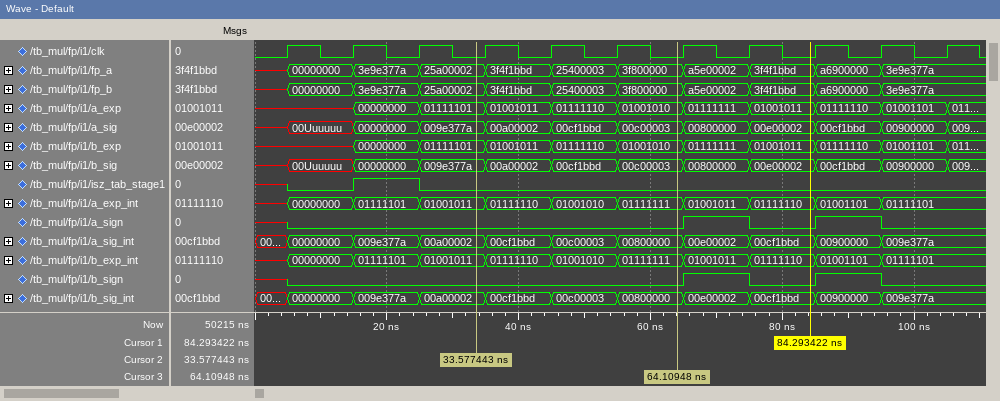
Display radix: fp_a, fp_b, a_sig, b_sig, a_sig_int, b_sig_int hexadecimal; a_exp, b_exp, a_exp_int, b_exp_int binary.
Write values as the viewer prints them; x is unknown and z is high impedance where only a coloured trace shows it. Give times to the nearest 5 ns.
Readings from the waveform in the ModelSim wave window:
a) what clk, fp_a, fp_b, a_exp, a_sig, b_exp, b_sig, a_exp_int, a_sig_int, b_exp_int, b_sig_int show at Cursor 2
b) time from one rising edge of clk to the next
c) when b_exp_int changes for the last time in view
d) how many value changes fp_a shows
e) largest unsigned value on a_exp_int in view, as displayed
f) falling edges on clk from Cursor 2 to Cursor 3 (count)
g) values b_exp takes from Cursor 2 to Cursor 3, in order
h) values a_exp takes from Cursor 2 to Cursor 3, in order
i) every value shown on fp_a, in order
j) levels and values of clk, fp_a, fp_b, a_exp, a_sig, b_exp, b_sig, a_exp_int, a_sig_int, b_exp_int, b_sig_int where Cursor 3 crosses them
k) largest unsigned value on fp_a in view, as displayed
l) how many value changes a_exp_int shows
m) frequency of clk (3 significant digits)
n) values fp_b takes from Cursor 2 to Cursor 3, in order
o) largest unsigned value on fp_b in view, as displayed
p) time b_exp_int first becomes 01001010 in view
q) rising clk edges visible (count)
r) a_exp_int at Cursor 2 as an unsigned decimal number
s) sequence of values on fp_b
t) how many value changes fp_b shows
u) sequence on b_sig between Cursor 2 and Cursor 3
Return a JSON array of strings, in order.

["clk=0, fp_a=25a00002, fp_b=25a00002, a_exp=01111101, a_sig=009e377a, b_exp=01111101, b_sig=009e377a, a_exp_int=01001011, a_sig_int=00a00002, b_exp_int=01001011, b_sig_int=00a00002", "10 ns", "95 ns", "10", "01111111", "3", "01111101, 01001011, 01111110, 01001010", "01111101, 01001011, 01111110, 01001010", "x, 00000000, 3e9e377a, 25a00002, 3f4f1bbd, 25400003, 3f800000, a5e00002, 3f4f1bbd, a6900000, 3e9e377a", "clk=0, fp_a=3f800000, fp_b=3f800000, a_exp=01001010, a_sig=00c00003, b_exp=01001010, b_sig=00c00003, a_exp_int=01111111, a_sig_int=00800000, b_exp_int=01111111, b_sig_int=00800000", "a6900000", "10", "100 MHz", "25a00002, 3f4f1bbd, 25400003, 3f800000", "a6900000", "45 ns", "11", "75", "x, 00000000, 3e9e377a, 25a00002, 3f4f1bbd, 25400003, 3f800000, a5e00002, 3f4f1bbd, a6900000, 3e9e377a", "10", "009e377a, 00a00002, 00cf1bbd, 00c00003"]
